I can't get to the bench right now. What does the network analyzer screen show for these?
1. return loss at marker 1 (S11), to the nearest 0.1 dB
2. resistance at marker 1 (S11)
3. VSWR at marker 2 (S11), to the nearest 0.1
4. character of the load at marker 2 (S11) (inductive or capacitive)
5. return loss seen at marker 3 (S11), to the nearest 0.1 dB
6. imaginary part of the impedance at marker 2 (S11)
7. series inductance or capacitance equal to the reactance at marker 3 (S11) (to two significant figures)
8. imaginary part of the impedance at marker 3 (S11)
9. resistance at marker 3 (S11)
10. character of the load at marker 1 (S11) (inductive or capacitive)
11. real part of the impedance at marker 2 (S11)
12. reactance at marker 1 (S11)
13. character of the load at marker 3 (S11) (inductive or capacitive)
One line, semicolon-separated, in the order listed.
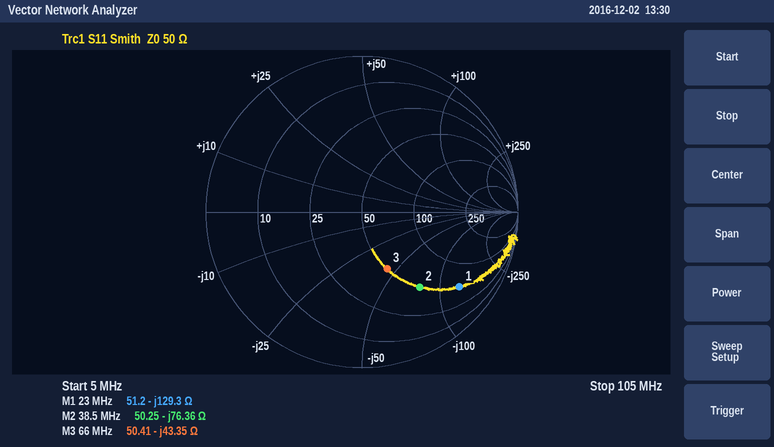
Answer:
2.1 dB; 51.2 Ω; 4.1; capacitive; 8.0 dB; -76.36 Ω; 56 pF; -43.35 Ω; 50.41 Ω; capacitive; 50.25 Ω; -129.3 Ω; capacitive
